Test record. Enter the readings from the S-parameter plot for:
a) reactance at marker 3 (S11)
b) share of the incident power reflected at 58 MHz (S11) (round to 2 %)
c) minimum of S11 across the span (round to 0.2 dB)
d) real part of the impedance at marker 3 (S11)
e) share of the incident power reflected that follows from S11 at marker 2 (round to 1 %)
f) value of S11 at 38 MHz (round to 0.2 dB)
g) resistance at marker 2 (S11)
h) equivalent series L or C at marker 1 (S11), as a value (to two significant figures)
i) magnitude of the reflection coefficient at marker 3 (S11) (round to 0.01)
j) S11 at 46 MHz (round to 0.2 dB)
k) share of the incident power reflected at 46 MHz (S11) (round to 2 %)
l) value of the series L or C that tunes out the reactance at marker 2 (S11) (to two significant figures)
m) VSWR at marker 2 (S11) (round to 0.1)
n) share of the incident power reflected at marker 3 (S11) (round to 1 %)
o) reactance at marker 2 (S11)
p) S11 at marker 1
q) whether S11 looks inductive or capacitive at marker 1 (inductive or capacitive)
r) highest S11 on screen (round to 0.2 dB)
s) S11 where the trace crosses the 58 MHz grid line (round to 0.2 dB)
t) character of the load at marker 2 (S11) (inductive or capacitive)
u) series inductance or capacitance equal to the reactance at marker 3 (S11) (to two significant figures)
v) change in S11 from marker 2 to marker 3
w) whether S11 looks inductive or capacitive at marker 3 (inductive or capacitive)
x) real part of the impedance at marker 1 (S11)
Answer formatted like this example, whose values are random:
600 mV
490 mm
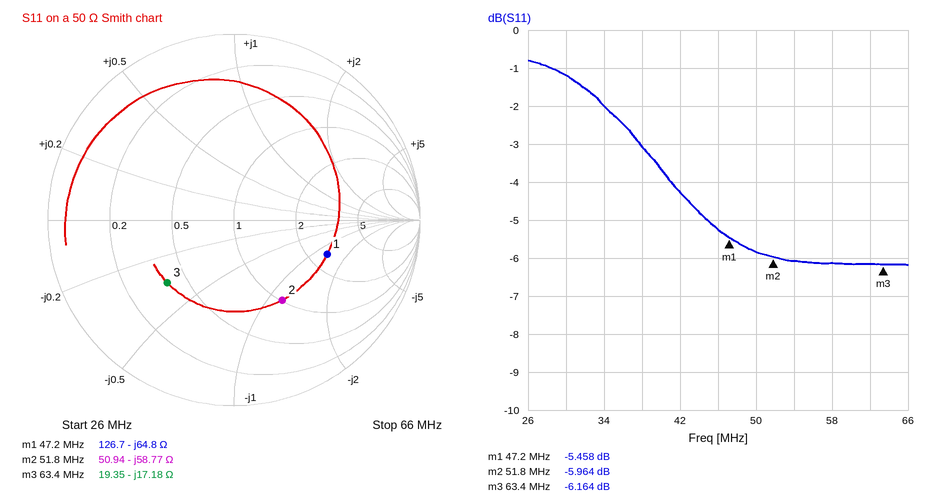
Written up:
-17.18 Ω
24 %
-6.2 dB
19.35 Ω
25 %
-3.0 dB
50.94 Ω
52 pF
0.49
-5.2 dB
30 %
180 nH
3.0
24 %
-58.77 Ω
-5.458 dB
capacitive
-0.8 dB
-6.2 dB
capacitive
150 pF
-0.200 dB
capacitive
126.7 Ω
